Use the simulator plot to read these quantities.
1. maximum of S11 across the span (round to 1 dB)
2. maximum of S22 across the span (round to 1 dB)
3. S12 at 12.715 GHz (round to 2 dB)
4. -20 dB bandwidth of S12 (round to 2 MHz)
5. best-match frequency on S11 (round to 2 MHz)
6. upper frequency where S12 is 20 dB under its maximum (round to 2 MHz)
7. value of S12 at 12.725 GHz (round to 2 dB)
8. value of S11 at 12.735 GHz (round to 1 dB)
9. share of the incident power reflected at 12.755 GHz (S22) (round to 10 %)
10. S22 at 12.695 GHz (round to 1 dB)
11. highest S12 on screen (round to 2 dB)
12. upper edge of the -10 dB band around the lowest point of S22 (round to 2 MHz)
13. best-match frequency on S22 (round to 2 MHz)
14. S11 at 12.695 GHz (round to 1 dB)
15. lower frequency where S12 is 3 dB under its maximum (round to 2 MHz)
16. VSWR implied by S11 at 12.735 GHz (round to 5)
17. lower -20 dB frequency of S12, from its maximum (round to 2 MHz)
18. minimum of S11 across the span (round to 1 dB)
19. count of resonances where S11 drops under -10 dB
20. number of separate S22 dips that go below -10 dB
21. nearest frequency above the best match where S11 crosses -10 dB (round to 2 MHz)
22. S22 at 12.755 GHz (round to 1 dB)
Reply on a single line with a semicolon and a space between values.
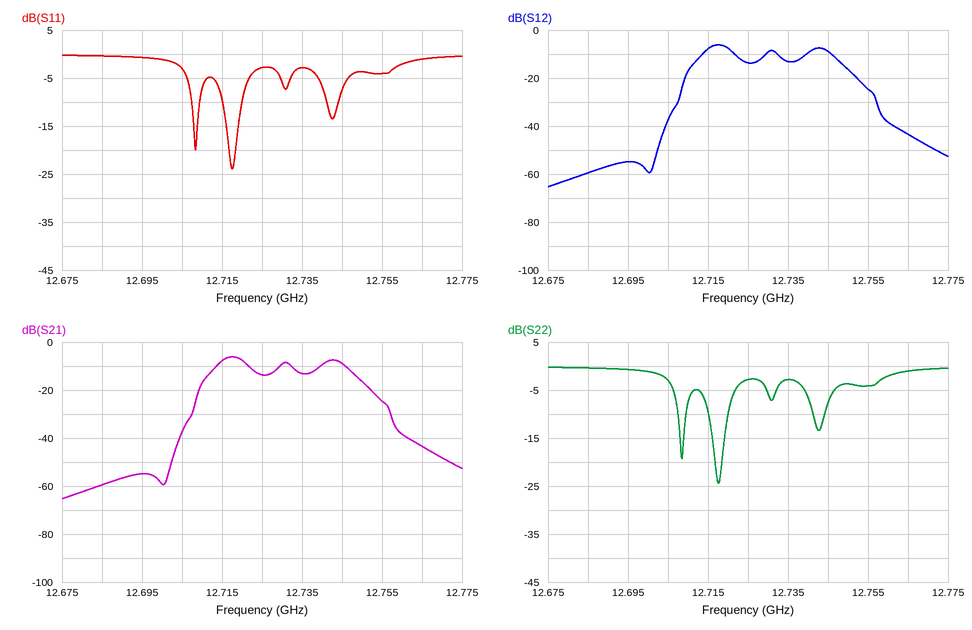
0 dB; 0 dB; -8 dB; 48 MHz; 12.718 GHz; 12.756 GHz; -14 dB; -3 dB; 40 %; -1 dB; -6 dB; 12.720 GHz; 12.718 GHz; -1 dB; 12.714 GHz; 5; 12.708 GHz; -24 dB; 3; 3; 12.720 GHz; -4 dB
